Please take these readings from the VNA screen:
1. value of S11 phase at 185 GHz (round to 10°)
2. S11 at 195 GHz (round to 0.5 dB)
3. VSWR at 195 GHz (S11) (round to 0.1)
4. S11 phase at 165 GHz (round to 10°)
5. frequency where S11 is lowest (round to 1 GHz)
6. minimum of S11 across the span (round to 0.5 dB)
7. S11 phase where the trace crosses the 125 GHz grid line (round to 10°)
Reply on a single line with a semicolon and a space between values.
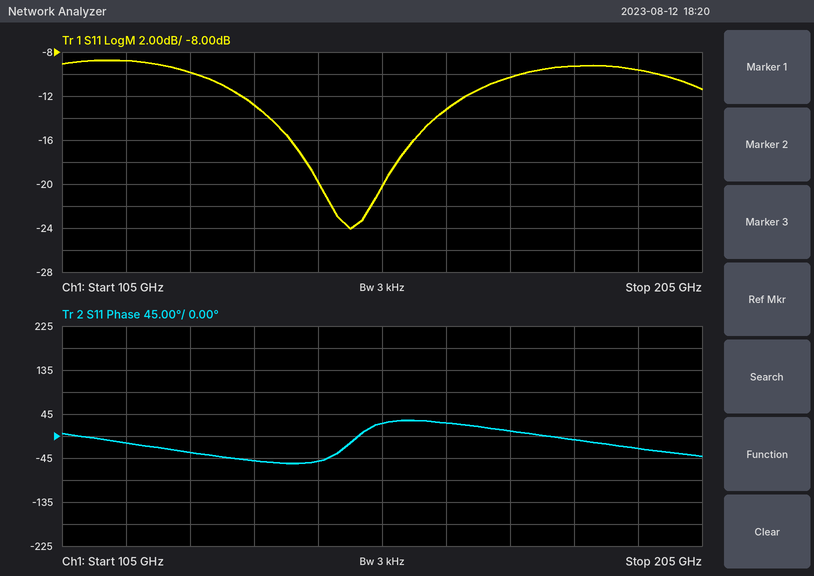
-10°; -9.5 dB; 2.0; 30°; 150 GHz; -24.0 dB; -30°
